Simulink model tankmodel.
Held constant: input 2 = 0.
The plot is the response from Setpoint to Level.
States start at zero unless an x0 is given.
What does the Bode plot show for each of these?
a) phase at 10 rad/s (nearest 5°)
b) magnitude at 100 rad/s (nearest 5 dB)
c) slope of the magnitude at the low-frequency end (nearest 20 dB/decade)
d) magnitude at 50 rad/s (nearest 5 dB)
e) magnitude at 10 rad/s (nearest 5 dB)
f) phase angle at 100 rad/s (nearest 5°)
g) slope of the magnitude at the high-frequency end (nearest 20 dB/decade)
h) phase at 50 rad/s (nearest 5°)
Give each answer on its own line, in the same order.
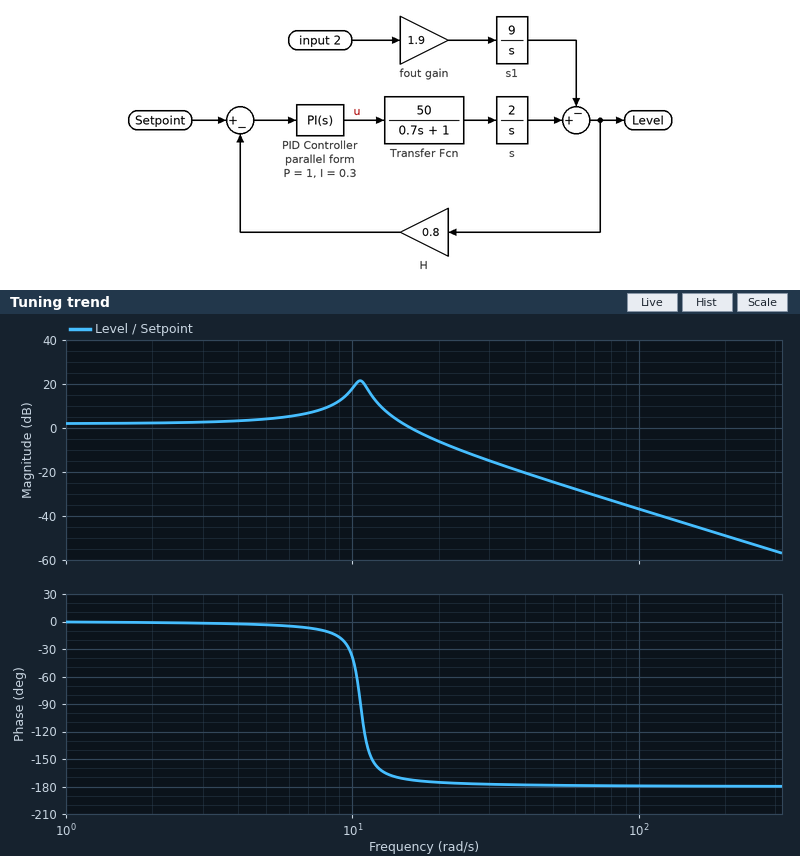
-40°
-35 dB
0 dB/decade
-25 dB
20 dB
-180°
-40 dB/decade
-180°
